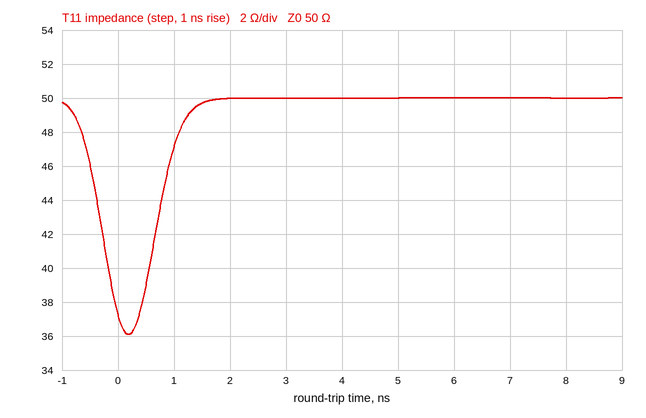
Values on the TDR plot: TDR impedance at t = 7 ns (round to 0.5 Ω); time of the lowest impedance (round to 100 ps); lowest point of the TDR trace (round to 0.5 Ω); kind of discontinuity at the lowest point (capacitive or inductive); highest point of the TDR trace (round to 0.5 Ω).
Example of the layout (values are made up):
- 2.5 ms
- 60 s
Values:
- 50.0 Ω
- 200 ps
- 36.0 Ω
- capacitive
- 50.0 Ω
